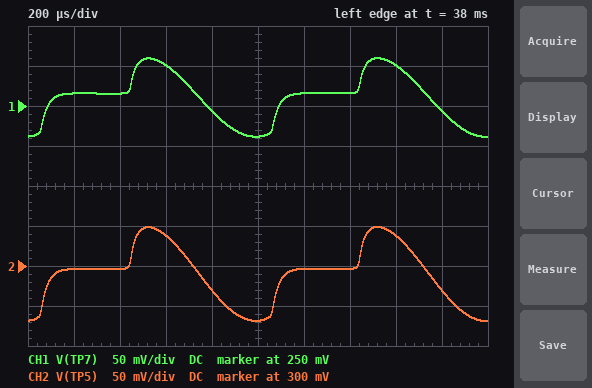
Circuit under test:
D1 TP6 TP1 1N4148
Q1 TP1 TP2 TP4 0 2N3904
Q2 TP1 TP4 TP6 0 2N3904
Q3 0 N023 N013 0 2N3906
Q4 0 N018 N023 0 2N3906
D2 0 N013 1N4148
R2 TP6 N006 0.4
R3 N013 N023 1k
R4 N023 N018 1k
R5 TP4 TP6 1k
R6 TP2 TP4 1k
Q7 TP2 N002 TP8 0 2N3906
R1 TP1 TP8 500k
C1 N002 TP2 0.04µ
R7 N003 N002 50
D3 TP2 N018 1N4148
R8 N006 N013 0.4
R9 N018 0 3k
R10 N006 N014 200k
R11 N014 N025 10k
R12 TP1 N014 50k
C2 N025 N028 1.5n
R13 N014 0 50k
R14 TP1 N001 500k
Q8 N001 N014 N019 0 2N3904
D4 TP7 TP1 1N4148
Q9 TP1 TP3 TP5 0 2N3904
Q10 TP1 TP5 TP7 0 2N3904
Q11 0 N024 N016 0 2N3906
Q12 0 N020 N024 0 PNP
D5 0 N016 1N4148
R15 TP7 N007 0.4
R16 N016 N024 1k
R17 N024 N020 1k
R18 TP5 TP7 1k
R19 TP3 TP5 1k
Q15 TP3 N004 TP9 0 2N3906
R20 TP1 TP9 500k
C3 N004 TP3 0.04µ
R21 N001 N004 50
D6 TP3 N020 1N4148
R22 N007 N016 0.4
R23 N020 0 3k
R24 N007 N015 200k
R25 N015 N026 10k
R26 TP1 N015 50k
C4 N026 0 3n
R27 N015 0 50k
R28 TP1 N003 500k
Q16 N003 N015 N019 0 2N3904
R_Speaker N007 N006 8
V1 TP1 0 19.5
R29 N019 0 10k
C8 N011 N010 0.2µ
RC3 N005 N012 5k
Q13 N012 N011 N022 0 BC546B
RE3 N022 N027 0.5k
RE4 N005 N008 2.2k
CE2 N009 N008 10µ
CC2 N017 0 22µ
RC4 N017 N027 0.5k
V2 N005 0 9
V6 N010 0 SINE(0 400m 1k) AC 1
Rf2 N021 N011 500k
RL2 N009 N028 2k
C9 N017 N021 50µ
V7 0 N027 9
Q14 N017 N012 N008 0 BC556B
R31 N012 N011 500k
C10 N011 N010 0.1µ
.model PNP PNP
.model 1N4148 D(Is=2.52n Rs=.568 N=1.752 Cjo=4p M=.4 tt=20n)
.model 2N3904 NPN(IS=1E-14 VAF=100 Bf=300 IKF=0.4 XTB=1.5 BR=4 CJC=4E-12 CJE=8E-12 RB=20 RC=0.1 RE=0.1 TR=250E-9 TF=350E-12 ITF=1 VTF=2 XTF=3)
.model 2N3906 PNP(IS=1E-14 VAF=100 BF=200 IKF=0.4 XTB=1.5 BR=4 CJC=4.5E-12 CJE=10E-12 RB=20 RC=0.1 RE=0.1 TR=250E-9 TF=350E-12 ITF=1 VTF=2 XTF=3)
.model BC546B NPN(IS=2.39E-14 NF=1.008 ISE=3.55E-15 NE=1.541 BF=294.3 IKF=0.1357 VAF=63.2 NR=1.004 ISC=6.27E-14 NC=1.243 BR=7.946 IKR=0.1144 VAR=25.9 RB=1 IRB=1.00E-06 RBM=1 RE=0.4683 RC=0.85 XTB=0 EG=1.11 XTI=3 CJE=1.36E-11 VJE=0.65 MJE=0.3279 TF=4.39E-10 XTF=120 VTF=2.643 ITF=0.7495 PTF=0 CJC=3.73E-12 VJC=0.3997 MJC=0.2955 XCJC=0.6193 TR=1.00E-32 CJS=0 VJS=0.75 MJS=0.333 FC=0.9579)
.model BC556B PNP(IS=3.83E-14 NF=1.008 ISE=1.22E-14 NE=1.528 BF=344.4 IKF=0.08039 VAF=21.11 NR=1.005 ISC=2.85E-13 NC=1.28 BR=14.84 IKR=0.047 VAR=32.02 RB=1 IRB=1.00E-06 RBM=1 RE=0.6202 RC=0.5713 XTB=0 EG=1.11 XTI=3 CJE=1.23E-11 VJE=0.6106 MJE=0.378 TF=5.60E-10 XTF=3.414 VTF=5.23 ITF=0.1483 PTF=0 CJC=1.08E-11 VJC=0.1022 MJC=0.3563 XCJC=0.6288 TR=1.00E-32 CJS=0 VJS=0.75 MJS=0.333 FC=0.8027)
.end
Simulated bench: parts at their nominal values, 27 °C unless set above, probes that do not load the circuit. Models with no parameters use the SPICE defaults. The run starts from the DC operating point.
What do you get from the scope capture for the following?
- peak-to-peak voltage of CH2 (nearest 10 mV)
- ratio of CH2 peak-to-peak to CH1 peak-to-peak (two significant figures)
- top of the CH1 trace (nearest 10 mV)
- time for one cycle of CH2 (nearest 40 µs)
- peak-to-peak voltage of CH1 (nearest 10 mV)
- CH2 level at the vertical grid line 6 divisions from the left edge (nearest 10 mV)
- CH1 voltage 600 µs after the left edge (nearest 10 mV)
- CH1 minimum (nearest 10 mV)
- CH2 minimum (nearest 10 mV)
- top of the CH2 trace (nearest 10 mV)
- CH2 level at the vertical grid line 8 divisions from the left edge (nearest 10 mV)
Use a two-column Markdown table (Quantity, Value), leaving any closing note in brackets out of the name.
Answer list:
| Quantity | Value |
|---|---|
| peak-to-peak voltage of CH2 | 120 mV |
| ratio of CH2 peak-to-peak to CH1 peak-to-peak | 1.2 |
| top of the CH1 trace | 310 mV |
| time for one cycle of CH2 | 1.00 ms |
| peak-to-peak voltage of CH1 | 100 mV |
| CH2 level at the vertical grid line 6 divisions from the left edge | 300 mV |
| CH1 voltage 600 µs after the left edge | 300 mV |
| CH1 minimum | 210 mV |
| CH2 minimum | 230 mV |
| top of the CH2 trace | 350 mV |
| CH2 level at the vertical grid line 8 divisions from the left edge | 340 mV |
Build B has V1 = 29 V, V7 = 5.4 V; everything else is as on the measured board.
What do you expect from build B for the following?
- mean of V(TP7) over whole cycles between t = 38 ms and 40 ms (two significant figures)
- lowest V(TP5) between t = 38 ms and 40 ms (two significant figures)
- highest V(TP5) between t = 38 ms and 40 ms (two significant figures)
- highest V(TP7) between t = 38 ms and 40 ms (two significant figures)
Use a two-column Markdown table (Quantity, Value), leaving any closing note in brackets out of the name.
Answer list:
| Quantity | Value |
|---|---|
| mean of V(TP7) over whole cycles between t = 38 ms and 40 ms | 380 mV |
| lowest V(TP5) between t = 38 ms and 40 ms | 370 mV |
| highest V(TP5) between t = 38 ms and 40 ms | 490 mV |
| highest V(TP7) between t = 38 ms and 40 ms | 430 mV |
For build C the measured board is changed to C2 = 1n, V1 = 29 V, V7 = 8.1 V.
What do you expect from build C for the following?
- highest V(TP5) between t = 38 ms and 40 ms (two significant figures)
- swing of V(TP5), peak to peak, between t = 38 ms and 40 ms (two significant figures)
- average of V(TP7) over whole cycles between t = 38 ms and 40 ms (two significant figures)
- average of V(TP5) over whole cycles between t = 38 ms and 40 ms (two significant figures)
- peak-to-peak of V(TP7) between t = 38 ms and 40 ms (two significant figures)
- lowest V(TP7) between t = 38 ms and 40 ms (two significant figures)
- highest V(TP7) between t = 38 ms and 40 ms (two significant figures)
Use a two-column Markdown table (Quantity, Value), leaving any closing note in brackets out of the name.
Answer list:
| Quantity | Value |
|---|---|
| highest V(TP5) between t = 38 ms and 40 ms | 470 mV |
| swing of V(TP5), peak to peak, between t = 38 ms and 40 ms | 79 mV |
| average of V(TP7) over whole cycles between t = 38 ms and 40 ms | 380 mV |
| average of V(TP5) over whole cycles between t = 38 ms and 40 ms | 430 mV |
| peak-to-peak of V(TP7) between t = 38 ms and 40 ms | 66 mV |
| lowest V(TP7) between t = 38 ms and 40 ms | 350 mV |
| highest V(TP7) between t = 38 ms and 40 ms | 420 mV |
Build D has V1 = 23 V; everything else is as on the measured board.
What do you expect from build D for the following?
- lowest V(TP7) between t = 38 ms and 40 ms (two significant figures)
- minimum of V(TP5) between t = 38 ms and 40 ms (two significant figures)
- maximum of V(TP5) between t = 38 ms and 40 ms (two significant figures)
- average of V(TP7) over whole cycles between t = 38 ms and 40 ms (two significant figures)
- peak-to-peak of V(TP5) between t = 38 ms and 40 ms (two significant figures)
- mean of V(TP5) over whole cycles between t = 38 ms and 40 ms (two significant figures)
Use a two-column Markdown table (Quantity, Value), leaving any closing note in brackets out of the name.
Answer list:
| Quantity | Value |
|---|---|
| lowest V(TP7) between t = 38 ms and 40 ms | 260 mV |
| minimum of V(TP5) between t = 38 ms and 40 ms | 280 mV |
| maximum of V(TP5) between t = 38 ms and 40 ms | 400 mV |
| average of V(TP7) over whole cycles between t = 38 ms and 40 ms | 310 mV |
| peak-to-peak of V(TP5) between t = 38 ms and 40 ms | 120 mV |
| mean of V(TP5) over whole cycles between t = 38 ms and 40 ms | 340 mV |
